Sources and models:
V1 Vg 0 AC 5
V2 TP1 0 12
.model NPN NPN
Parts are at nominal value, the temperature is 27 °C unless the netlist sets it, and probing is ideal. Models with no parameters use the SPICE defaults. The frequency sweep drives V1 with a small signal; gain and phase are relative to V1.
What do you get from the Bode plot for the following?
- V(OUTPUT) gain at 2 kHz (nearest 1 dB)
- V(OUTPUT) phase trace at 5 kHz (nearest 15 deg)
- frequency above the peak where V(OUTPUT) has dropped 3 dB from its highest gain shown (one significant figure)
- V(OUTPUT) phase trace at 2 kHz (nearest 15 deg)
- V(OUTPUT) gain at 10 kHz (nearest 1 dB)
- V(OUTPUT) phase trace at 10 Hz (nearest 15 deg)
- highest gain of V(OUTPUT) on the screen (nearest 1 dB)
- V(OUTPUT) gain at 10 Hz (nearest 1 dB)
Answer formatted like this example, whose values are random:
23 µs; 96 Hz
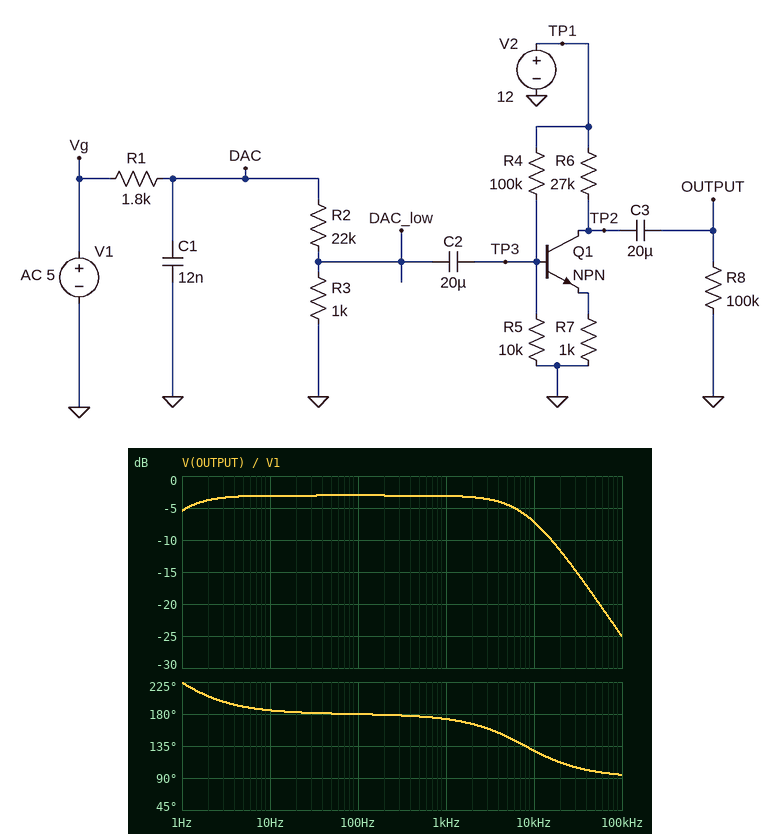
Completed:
-3 dB; 150 deg; 8 kHz; 165 deg; -7 dB; 180 deg; -3 dB; -3 dB
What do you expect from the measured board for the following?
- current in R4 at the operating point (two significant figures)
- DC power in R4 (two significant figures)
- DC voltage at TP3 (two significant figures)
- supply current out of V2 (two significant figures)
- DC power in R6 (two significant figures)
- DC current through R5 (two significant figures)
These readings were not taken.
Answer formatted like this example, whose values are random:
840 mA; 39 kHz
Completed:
110 µA; 1.2 mW; 1.1 V; 420 µA; 2.7 mW; 110 µA
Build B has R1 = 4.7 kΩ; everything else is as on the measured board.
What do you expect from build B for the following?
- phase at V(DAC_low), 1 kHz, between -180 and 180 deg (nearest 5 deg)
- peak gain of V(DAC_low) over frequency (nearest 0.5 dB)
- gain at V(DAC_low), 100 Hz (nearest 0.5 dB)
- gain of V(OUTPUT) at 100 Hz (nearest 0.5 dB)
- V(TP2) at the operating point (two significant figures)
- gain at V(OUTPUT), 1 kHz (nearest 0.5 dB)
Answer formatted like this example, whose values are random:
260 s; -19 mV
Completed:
-15 deg; -29.0 dB; -30.0 dB; -4.0 dB; 3.5 V; -4.5 dB
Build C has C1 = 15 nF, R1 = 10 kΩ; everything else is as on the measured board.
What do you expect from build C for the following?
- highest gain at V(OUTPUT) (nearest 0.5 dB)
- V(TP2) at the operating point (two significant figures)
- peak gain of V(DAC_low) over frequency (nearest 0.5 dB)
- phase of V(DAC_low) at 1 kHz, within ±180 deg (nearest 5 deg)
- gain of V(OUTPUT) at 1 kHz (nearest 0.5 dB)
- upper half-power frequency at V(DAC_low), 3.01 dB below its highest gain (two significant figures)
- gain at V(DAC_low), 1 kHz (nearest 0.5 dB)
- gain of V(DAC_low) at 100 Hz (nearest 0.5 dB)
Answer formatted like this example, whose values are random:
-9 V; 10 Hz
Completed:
-5.5 dB; 3.5 V; -30.5 dB; -35 deg; -7.0 dB; 1.2 kHz; -33.0 dB; -31.5 dB
